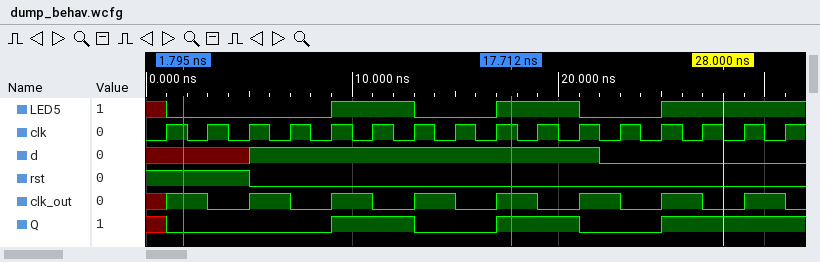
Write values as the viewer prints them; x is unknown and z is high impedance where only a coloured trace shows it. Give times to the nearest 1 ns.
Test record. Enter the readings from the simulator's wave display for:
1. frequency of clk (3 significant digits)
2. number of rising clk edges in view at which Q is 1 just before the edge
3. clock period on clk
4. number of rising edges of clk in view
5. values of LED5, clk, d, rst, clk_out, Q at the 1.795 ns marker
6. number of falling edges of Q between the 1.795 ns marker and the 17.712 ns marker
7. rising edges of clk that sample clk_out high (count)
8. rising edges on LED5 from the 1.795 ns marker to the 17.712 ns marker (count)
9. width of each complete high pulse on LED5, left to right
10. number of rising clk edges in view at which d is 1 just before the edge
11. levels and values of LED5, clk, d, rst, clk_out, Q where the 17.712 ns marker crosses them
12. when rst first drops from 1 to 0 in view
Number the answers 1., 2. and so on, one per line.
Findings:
1. 500 MHz
2. 7
3. 2 ns
4. 16
5. LED5=0, clk=1, d=x, rst=1, clk_out=1, Q=0
6. 1
7. 8
8. 2
9. 4 ns, 4 ns
10. 8
11. LED5=1, clk=1, d=1, rst=0, clk_out=1, Q=1
12. 5 ns
